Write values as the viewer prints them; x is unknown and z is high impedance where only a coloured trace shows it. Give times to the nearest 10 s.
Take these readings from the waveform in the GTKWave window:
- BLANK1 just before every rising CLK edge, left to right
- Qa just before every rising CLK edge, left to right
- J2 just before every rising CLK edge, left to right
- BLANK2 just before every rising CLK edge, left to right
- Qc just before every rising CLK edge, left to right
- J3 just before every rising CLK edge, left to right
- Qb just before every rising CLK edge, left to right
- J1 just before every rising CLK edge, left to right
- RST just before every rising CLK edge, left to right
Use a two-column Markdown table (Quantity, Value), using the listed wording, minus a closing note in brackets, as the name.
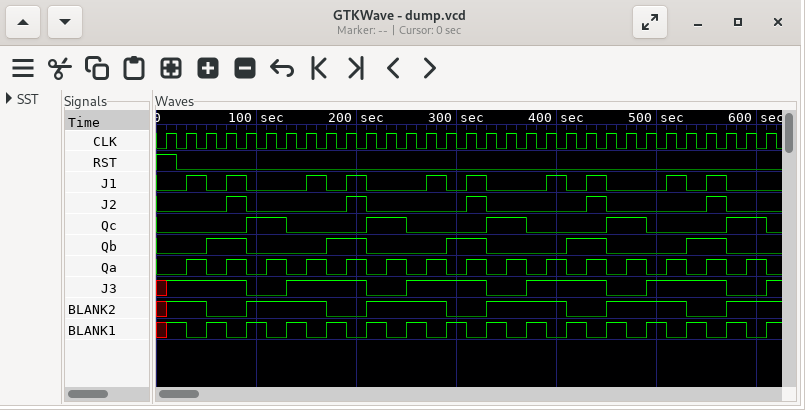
| Quantity | Value |
|---|---|
| BLANK1 just before every rising CLK edge, left to right | x 1 0 1 0 1 0 1 0 1 0 1 0 1 0 1 0 1 0 1 0 1 0 1 0 1 0 1 0 1 0 |
| Qa just before every rising CLK edge, left to right | 0 0 1 0 1 0 1 0 1 0 1 0 1 0 1 0 1 0 1 0 1 0 1 0 1 0 1 0 1 0 1 |
| J2 just before every rising CLK edge, left to right | 0 0 0 0 1 0 0 0 0 0 1 0 0 0 0 0 1 0 0 0 0 0 1 0 0 0 0 0 1 0 0 |
| BLANK2 just before every rising CLK edge, left to right | x 1 1 0 0 1 1 1 1 0 0 1 1 1 1 0 0 1 1 1 1 0 0 1 1 1 1 0 0 1 1 |
| Qc just before every rising CLK edge, left to right | 0 0 0 0 0 1 1 0 0 0 0 1 1 0 0 0 0 1 1 0 0 0 0 1 1 0 0 0 0 1 1 |
| J3 just before every rising CLK edge, left to right | x 1 1 1 1 0 0 1 1 1 1 0 0 1 1 1 1 0 0 1 1 1 1 0 0 1 1 1 1 0 0 |
| Qb just before every rising CLK edge, left to right | 0 0 0 1 1 0 0 0 0 1 1 0 0 0 0 1 1 0 0 0 0 1 1 0 0 0 0 1 1 0 0 |
| J1 just before every rising CLK edge, left to right | 0 0 1 0 1 0 0 0 1 0 1 0 0 0 1 0 1 0 0 0 1 0 1 0 0 0 1 0 1 0 0 |
| RST just before every rising CLK edge, left to right | 1 0 0 0 0 0 0 0 0 0 0 0 0 0 0 0 0 0 0 0 0 0 0 0 0 0 0 0 0 0 0 |
